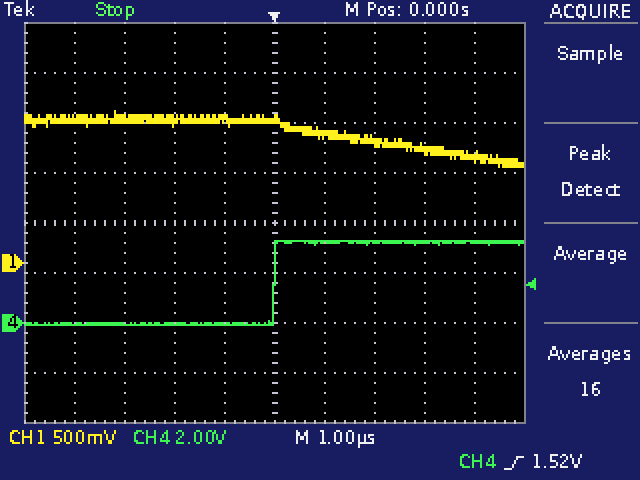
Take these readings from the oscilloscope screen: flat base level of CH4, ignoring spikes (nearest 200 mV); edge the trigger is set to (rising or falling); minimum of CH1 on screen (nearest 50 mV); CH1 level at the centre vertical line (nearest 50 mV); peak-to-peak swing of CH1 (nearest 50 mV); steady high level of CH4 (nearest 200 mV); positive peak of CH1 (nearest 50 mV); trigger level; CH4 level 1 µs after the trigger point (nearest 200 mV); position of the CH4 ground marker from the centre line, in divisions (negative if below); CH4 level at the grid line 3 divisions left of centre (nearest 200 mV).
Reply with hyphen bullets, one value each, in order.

- 0.0 V
- rising
- 950 mV
- 1.45 V
- 550 mV
- 3.2 V
- 1.50 V
- 1.52 V
- 3.2 V
- -2.0 div
- 0.0 V
